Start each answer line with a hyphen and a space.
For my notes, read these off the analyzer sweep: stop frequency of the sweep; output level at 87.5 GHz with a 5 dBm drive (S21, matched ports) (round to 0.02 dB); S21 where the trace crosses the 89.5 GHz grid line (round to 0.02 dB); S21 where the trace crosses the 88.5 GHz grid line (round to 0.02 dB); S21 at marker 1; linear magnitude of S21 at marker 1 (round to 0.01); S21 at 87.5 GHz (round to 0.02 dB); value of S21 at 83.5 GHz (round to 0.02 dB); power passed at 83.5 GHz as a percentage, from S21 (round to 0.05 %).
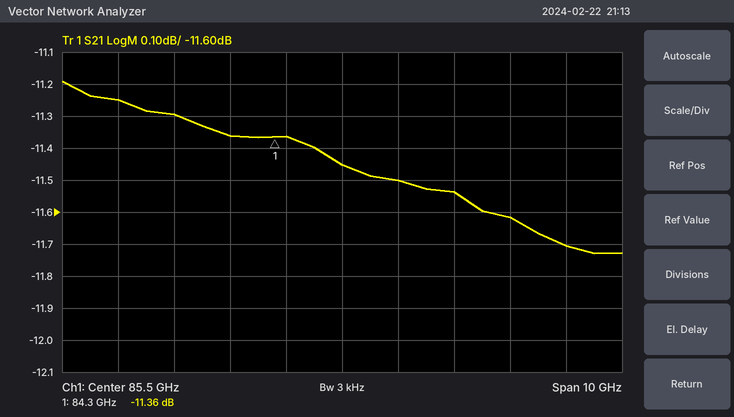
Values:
- 90.5 GHz
- -6.54 dBm
- -11.70 dB
- -11.62 dB
- -11.36 dB
- 0.27
- -11.54 dB
- -11.36 dB
- 7.30 %
